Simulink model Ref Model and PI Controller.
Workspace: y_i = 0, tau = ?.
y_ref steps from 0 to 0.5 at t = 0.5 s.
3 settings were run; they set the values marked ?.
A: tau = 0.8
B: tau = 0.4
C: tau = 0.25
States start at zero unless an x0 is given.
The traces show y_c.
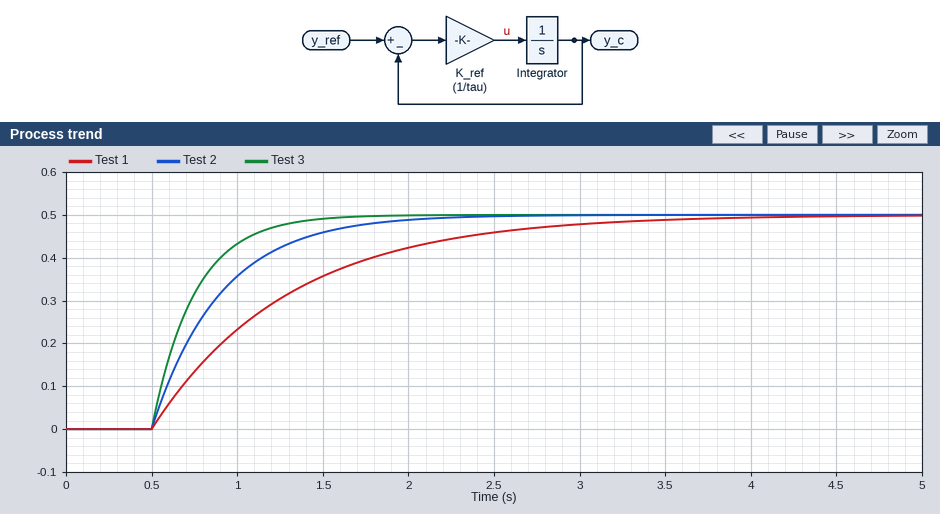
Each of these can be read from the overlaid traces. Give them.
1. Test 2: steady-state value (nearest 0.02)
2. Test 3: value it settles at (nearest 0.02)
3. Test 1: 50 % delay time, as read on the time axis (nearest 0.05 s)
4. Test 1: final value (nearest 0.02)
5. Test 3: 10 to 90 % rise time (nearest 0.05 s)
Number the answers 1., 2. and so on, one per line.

1. 0.50
2. 0.50
3. 1.05 s
4. 0.50
5. 0.55 s
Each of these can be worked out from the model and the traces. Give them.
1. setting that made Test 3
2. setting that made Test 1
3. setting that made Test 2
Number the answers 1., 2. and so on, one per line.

1. C
2. A
3. B
